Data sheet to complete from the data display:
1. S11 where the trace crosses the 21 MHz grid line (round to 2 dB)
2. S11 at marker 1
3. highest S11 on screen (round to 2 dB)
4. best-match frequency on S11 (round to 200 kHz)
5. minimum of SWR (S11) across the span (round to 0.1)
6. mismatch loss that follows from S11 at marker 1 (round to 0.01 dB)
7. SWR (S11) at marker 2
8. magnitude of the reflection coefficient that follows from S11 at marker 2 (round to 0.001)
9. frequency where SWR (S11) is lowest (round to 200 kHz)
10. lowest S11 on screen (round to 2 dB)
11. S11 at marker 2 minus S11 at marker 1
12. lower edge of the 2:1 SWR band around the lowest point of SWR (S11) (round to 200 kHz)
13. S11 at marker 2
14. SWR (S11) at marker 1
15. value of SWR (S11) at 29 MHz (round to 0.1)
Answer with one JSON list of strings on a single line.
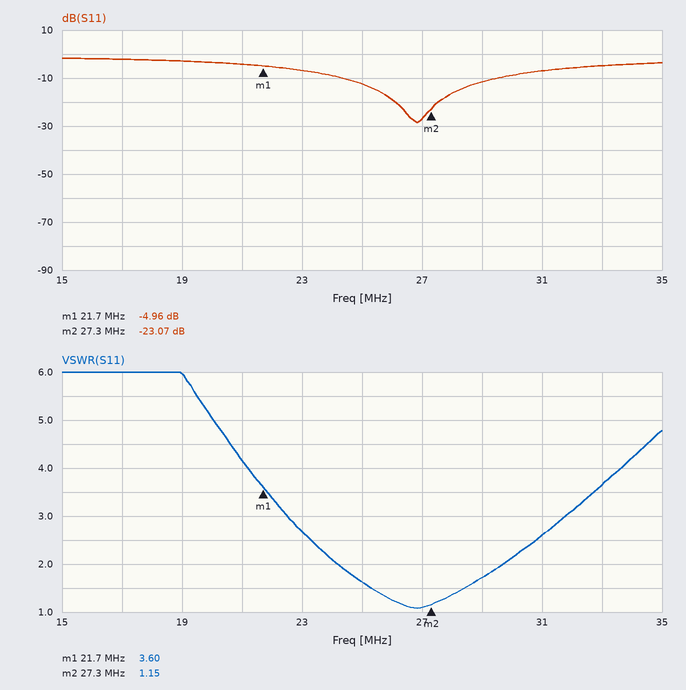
["-4 dB", "-4.96 dB", "-2 dB", "26.8 MHz", "1.1", "1.67 dB", "1.15", "0.070", "26.8 MHz", "-28 dB", "-18.11 dB", "24.2 MHz", "-23.07 dB", "3.60", "1.7"]
